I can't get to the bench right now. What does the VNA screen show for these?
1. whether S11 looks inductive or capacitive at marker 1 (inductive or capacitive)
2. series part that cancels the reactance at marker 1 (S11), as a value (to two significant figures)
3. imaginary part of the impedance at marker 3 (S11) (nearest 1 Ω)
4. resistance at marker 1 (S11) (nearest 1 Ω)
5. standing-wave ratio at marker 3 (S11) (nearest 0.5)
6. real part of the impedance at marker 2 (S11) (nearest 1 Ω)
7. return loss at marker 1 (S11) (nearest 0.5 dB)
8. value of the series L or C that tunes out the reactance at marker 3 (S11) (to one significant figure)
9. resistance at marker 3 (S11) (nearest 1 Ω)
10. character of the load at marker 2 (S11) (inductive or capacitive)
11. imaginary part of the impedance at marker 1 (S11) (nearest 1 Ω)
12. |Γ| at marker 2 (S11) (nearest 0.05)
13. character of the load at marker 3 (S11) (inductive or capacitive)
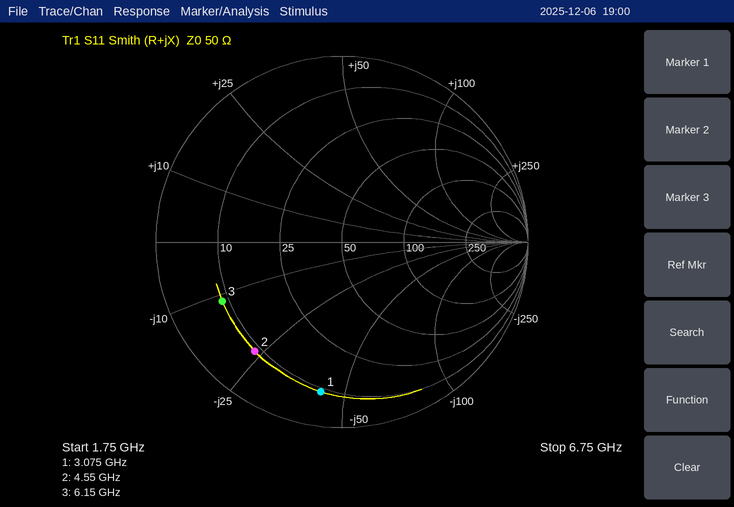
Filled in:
capacitive
2.2 nH
-11 Ω
9 Ω
6.0
9 Ω
2.0 dB
300 pH
9 Ω
capacitive
-43 Ω
0.75
capacitive
